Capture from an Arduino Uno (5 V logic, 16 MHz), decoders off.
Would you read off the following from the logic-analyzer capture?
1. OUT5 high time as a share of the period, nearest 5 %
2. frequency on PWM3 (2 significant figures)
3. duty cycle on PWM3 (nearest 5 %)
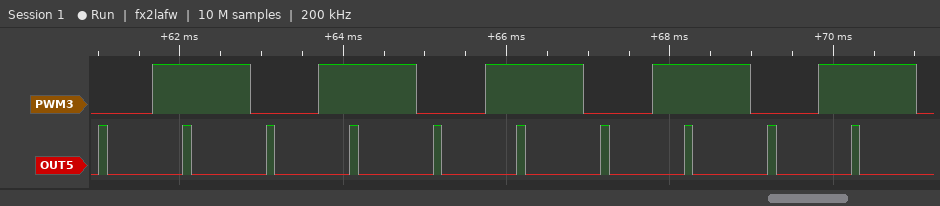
10 %
490 Hz
60 %
